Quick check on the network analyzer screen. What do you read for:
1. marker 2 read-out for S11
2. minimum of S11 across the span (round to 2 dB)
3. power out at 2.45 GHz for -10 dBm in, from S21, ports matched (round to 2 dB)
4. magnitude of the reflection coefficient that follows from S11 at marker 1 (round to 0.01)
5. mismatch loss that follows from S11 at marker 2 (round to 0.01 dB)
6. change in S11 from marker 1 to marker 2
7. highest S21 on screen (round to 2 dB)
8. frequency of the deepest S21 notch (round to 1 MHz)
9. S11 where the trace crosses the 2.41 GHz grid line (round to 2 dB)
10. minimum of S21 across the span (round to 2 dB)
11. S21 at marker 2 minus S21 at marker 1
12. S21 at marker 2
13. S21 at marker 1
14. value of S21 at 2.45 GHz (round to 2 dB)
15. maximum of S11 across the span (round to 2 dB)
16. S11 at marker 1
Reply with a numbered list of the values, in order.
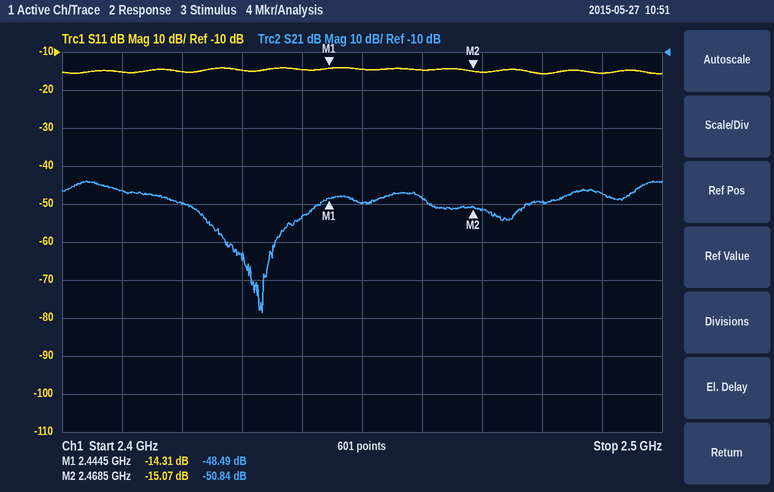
1. -15.07 dB
2. -16 dB
3. -60 dBm
4. 0.19
5. 0.14 dB
6. -0.76 dB
7. -44 dB
8. 2.433 GHz
9. -16 dB
10. -78 dB
11. -2.35 dB
12. -50.84 dB
13. -48.49 dB
14. -50 dB
15. -14 dB
16. -14.31 dB
